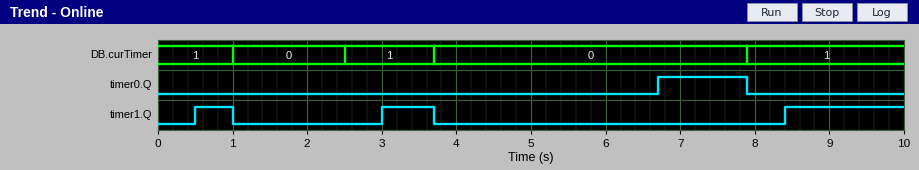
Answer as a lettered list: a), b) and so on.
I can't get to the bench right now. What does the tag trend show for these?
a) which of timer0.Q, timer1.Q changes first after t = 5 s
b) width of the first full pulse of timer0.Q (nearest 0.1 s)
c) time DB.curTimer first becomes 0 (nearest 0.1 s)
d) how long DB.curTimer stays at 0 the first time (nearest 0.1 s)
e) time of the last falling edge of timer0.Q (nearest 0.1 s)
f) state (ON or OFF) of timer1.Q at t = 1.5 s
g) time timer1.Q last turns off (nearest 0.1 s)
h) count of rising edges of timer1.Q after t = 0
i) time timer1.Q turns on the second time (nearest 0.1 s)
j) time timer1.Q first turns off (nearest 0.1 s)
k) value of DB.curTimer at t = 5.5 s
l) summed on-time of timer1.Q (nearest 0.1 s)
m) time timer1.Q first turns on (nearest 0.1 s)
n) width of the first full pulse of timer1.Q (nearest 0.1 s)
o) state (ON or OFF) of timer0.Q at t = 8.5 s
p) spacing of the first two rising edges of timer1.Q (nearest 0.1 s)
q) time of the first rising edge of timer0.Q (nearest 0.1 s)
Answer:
a) timer0.Q
b) 1.2 s
c) 1.0 s
d) 1.5 s
e) 7.9 s
f) OFF
g) 3.7 s
h) 3
i) 3.0 s
j) 1.0 s
k) 0
l) 2.8 s
m) 0.5 s
n) 0.5 s
o) OFF
p) 2.5 s
q) 6.7 s
